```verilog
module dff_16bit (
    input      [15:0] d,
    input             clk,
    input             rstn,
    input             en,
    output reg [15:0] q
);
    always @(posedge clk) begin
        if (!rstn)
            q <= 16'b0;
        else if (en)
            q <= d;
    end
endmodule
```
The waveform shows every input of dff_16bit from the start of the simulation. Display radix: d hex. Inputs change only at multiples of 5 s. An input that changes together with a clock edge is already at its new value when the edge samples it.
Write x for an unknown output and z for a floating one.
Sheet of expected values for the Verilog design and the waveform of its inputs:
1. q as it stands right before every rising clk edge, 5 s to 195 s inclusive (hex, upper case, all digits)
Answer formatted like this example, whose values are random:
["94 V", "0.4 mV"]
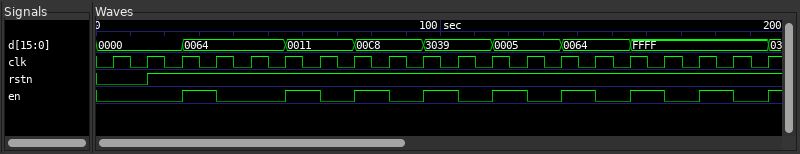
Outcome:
["x, 0000, 0000, 0064, 0064, 0064, 0011, 0011, 00C8, 00C8, 3039, 3039, 0005, 0005, 0064, 0064, FFFF, FFFF, FFFF, FFFF"]
